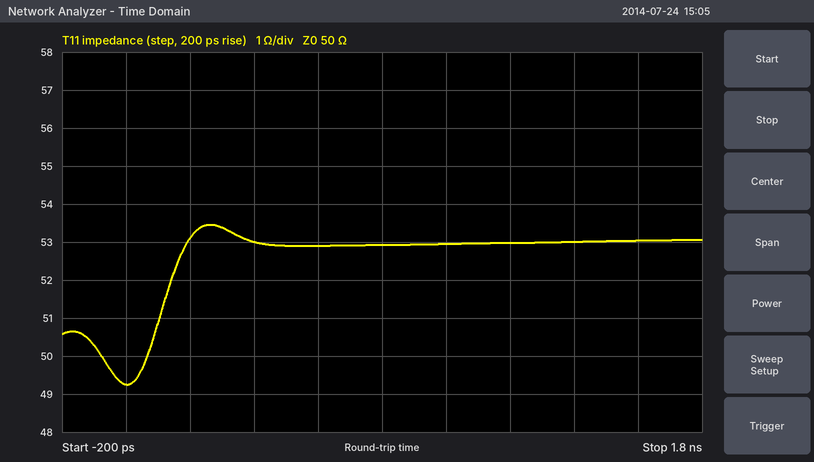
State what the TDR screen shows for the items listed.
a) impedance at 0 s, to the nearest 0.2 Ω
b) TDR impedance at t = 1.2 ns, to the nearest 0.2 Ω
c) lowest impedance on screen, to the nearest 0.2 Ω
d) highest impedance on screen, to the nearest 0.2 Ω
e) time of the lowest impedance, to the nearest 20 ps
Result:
49.2 Ω
53.0 Ω
49.2 Ω
53.4 Ω
0 ps
